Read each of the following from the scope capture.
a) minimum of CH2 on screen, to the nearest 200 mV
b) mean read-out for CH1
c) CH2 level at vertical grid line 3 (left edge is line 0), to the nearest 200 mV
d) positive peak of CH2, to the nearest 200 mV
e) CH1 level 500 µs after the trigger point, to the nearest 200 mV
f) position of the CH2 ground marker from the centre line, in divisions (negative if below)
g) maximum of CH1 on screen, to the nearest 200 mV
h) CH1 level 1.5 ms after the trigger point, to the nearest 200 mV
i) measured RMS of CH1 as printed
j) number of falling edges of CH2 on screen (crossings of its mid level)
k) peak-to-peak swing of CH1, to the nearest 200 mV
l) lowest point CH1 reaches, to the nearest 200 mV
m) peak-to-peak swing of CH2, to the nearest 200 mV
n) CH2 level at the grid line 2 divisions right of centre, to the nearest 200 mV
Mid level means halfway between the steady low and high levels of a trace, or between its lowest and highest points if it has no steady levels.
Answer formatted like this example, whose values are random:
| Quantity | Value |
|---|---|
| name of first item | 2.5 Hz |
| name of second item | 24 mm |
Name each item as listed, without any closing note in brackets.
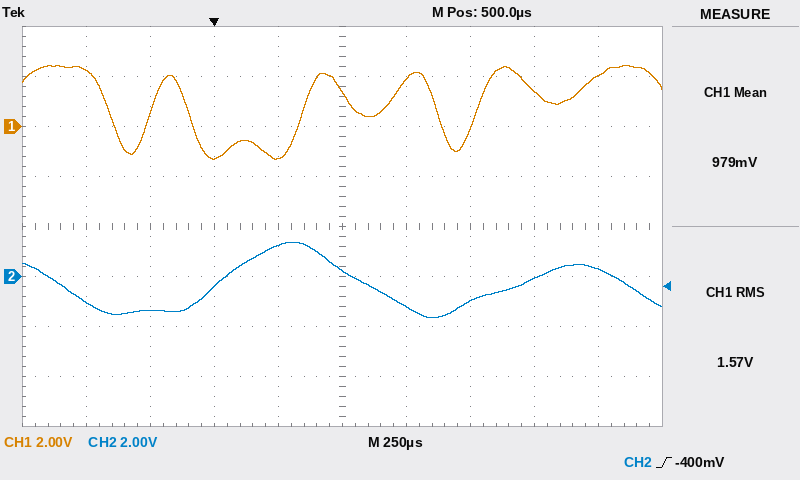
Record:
| Quantity | Value |
|---|---|
| minimum of CH2 on screen, to the nearest 200 mV | -1.6 V |
| mean read-out for CH1 | 979 mV |
| CH2 level at vertical grid line 3 (left edge is line 0), to the nearest 200 mV | -400 mV |
| positive peak of CH2, to the nearest 200 mV | 1.4 V |
| CH1 level 500 µs after the trigger point, to the nearest 200 mV | 1.4 V |
| position of the CH2 ground marker from the centre line, in divisions | -1.0 div |
| maximum of CH1 on screen, to the nearest 200 mV | 2.4 V |
| CH1 level 1.5 ms after the trigger point, to the nearest 200 mV | 2.0 V |
| measured RMS of CH1 as printed | 1.57 V |
| number of falling edges of CH2 on screen | 3 |
| peak-to-peak swing of CH1, to the nearest 200 mV | 3.8 V |
| lowest point CH1 reaches, to the nearest 200 mV | -1.4 V |
| peak-to-peak swing of CH2, to the nearest 200 mV | 3.0 V |
| CH2 level at the grid line 2 divisions right of centre, to the nearest 200 mV | -1.0 V |
